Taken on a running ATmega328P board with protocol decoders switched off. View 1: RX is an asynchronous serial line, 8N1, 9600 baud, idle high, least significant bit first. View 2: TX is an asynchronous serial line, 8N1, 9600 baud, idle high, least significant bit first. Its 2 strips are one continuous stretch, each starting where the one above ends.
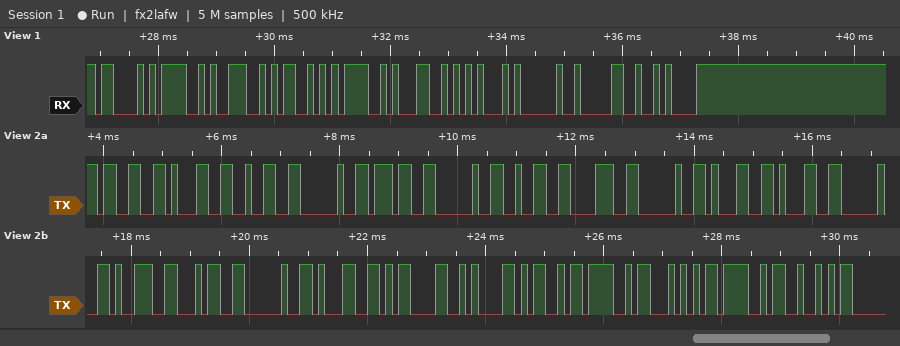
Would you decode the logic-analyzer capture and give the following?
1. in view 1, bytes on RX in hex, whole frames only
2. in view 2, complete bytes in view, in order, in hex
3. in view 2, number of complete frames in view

0x43 0x4F 0x4E 0x53 0x4F 0x4C 0x45 0x20 0x30 0x0A
33 31 32 20 37 20 32 38 20 31 31 20 39 34 20 31 0D 0A 4D 4F 54 4F 52
23
